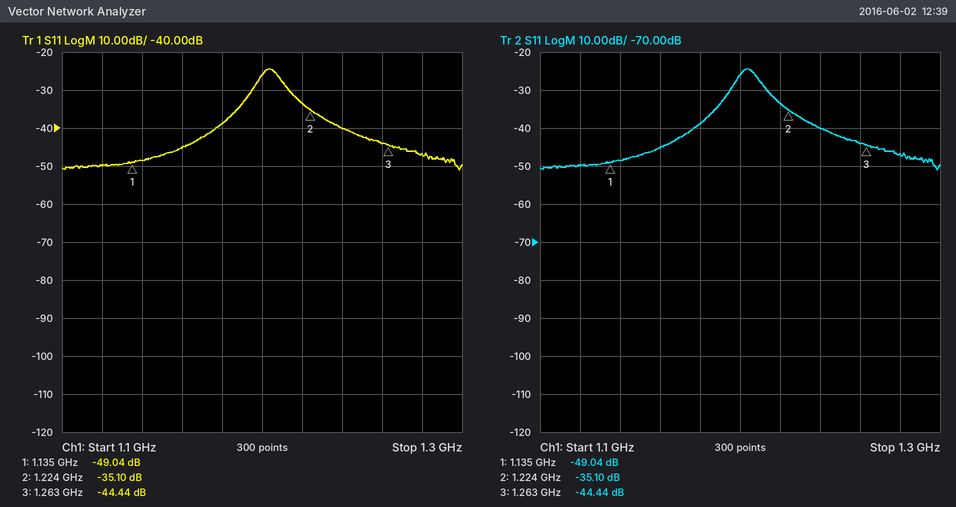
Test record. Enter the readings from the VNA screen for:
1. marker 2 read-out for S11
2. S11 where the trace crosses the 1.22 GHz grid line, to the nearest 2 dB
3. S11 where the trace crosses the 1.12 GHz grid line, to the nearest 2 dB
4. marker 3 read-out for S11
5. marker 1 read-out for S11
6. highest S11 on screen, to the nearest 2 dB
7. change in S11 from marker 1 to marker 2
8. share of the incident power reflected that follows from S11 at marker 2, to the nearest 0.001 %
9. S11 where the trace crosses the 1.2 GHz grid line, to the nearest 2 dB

-35.10 dB
-34 dB
-50 dB
-44.44 dB
-49.04 dB
-24 dB
13.94 dB
0.031 %
-26 dB
